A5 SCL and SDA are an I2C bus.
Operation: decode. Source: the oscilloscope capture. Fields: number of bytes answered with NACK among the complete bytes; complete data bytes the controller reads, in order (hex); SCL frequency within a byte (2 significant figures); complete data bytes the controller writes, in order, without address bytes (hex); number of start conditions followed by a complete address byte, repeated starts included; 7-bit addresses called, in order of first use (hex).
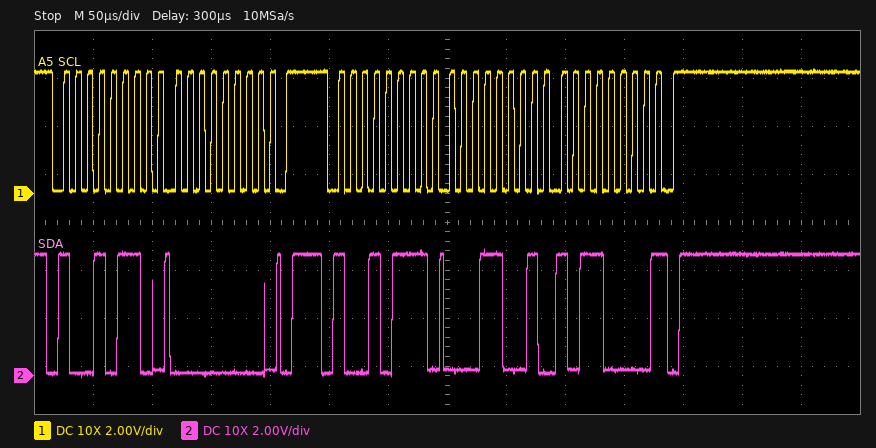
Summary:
1
19 B0
100 kHz
00
2
0x4B
